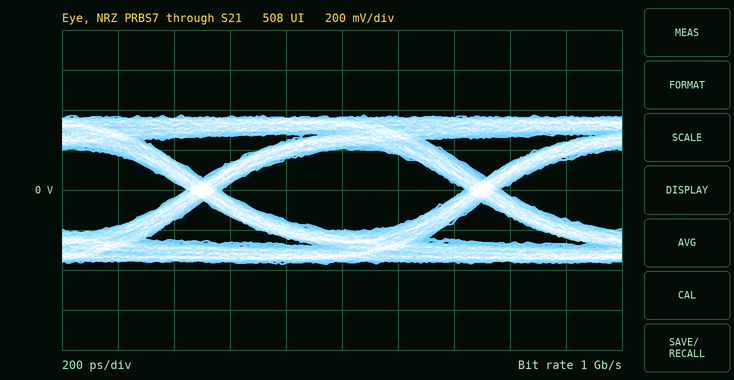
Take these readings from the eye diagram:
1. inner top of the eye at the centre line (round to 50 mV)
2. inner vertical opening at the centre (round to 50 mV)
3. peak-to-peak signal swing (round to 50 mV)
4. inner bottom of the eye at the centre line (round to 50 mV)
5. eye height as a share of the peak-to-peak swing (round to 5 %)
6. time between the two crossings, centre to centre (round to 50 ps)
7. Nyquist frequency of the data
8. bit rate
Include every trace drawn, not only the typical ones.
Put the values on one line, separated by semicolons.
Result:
200 mV; 400 mV; 750 mV; -200 mV; 55 %; 1.00 ns; 500 MHz; 1 Gb/s
